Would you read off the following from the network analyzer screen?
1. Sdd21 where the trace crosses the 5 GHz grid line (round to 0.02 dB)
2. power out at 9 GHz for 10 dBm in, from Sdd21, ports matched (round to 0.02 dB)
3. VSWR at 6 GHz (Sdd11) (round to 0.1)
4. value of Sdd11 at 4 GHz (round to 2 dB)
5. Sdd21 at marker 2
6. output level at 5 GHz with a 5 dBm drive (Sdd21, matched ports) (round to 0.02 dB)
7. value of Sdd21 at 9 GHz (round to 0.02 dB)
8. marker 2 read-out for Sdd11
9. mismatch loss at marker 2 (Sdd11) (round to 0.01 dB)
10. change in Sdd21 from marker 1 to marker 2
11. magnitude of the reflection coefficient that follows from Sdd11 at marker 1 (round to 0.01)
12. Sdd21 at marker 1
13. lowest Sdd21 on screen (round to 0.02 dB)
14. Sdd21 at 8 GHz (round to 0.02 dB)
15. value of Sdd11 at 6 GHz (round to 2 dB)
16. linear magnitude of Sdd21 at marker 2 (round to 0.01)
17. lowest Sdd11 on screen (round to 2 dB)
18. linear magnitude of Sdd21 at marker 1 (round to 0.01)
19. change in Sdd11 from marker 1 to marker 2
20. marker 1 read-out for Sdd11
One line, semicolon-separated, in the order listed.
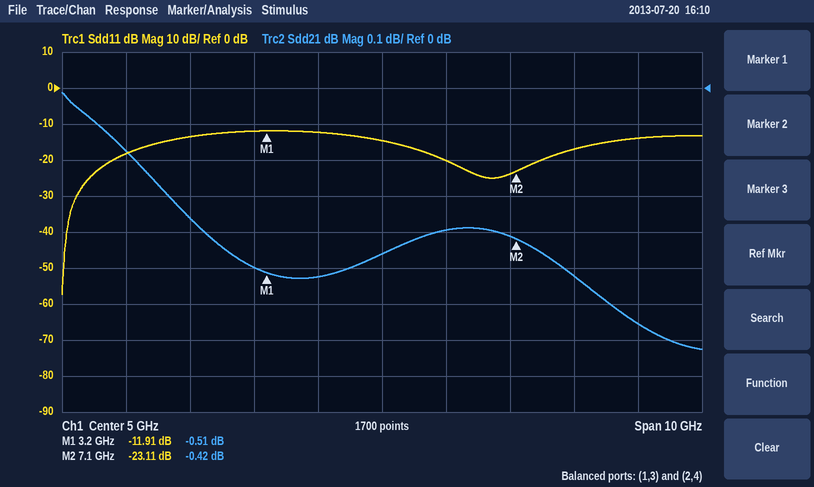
-0.46 dB; 9.34 dBm; 1.2; -12 dB; -0.42 dB; 4.54 dBm; -0.66 dB; -23.11 dB; 0.02 dB; 0.09 dB; 0.25; -0.51 dB; -0.72 dB; -0.52 dB; -20 dB; 0.95; -58 dB; 0.94; -11.20 dB; -11.91 dB
